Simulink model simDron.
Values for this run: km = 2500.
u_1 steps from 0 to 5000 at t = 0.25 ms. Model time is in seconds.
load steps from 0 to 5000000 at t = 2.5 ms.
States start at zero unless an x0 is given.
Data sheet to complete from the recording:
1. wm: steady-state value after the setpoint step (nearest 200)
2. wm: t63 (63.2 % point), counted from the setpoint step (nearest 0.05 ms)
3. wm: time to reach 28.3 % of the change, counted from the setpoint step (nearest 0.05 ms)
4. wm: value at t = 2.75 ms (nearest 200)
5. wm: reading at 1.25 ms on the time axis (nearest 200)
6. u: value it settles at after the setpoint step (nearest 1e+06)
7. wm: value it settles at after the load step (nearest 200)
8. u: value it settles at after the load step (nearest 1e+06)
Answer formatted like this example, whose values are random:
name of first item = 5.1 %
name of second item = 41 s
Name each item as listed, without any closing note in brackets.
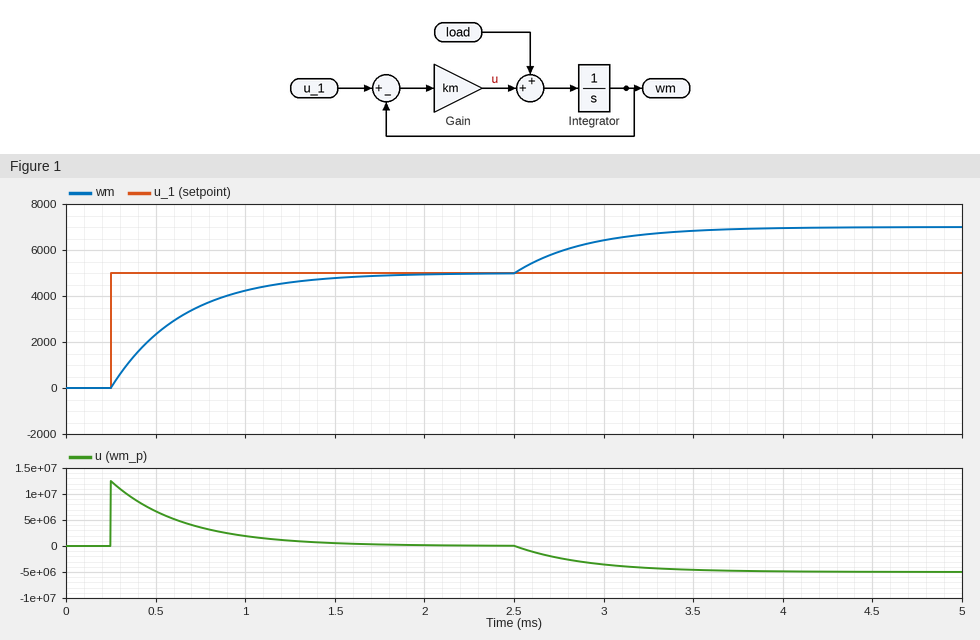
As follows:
wm: steady-state value after the setpoint step = 5000
wm: t63 (63.2 % point), counted from the setpoint step = 0.40 ms
wm: time to reach 28.3 % of the change, counted from the setpoint step = 0.15 ms
wm: value at t = 2.75 ms = 6000
wm: reading at 1.25 ms on the time axis = 4600
u: value it settles at after the setpoint step = 0
wm: value it settles at after the load step = 7000
u: value it settles at after the load step = -5000000
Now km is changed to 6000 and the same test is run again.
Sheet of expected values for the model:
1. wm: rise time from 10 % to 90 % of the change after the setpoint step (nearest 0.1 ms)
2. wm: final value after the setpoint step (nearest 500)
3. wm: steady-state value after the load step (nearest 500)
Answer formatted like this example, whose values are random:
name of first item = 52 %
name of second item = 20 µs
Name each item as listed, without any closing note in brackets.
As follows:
wm: rise time from 10 % to 90 % of the change after the setpoint step = 0.4 ms
wm: final value after the setpoint step = 5000
wm: steady-state value after the load step = 6000
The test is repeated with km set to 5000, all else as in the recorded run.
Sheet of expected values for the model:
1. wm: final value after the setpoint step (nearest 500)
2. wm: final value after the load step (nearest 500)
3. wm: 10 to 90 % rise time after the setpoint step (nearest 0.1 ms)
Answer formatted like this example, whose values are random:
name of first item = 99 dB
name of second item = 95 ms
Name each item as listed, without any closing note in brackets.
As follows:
wm: final value after the setpoint step = 5000
wm: final value after the load step = 6000
wm: 10 to 90 % rise time after the setpoint step = 0.4 ms
